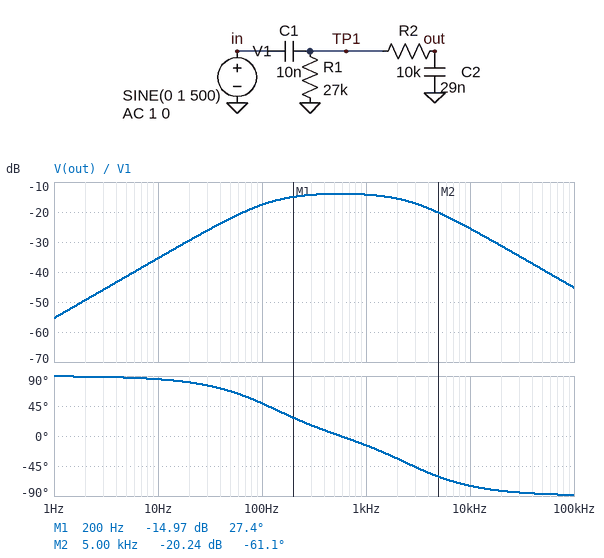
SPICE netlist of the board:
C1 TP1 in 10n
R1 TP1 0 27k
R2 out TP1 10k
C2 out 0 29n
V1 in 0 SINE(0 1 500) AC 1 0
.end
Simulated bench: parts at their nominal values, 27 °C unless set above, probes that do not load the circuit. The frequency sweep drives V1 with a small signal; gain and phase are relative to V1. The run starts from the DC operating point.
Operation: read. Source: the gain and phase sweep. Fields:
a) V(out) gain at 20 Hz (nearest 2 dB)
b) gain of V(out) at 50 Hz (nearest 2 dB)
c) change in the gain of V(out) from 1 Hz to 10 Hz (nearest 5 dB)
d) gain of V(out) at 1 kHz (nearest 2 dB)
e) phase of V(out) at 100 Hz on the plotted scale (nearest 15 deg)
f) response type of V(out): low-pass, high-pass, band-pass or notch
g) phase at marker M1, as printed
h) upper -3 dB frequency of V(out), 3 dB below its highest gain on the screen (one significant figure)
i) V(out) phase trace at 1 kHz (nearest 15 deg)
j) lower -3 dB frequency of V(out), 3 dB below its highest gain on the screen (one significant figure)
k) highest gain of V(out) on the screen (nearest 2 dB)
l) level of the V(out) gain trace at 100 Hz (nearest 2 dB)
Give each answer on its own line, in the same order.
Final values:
-30 dB
-22 dB
20 dB
-14 dB
45 deg
band-pass
27.4 deg
3 kHz
-15 deg
100 Hz
-14 dB
-18 dB
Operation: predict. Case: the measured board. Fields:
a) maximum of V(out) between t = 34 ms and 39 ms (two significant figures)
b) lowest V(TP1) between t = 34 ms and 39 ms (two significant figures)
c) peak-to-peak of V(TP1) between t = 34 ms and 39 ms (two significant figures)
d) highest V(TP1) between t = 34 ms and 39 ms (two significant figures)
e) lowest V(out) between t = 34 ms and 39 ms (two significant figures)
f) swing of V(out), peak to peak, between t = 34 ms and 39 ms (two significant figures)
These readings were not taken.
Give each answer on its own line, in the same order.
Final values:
200 mV
-270 mV
540 mV
270 mV
-200 mV
400 mV
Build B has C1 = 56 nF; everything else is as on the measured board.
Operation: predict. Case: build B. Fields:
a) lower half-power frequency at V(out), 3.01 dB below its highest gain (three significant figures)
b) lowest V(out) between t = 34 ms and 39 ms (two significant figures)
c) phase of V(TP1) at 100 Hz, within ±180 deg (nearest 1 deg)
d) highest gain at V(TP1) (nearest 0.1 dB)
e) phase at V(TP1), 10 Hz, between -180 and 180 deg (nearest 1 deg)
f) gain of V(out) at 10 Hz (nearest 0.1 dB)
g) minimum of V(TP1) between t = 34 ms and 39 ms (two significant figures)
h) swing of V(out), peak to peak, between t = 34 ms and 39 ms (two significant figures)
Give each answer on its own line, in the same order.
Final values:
58.0 Hz
-540 mV
37 deg
0 dB
82 deg
-20.5 dB
-730 mV
1.1 V
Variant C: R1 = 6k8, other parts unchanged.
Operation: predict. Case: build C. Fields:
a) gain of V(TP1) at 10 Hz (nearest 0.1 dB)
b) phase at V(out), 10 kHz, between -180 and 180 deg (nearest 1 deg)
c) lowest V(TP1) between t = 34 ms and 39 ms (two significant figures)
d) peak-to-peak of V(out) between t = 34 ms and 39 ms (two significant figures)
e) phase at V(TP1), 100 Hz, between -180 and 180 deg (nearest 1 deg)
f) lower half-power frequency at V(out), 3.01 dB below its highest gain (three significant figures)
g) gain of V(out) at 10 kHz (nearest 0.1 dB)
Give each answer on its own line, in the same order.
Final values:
-47.4 dB
-66 deg
-150 mV
220 mV
81 deg
270 Hz
-25.9 dB
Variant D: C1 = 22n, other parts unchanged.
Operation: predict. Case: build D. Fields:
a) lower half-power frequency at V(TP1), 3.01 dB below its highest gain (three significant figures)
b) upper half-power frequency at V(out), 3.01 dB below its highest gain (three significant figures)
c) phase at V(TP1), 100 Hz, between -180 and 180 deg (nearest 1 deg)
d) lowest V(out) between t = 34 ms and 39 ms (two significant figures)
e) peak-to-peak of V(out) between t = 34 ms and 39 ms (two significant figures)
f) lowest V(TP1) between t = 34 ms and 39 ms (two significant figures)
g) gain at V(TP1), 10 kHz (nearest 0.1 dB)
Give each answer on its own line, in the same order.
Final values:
1.22 kHz
1.63 kHz
52 deg
-350 mV
710 mV
-480 mV
-0.1 dB
